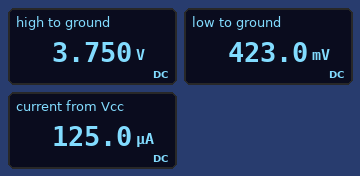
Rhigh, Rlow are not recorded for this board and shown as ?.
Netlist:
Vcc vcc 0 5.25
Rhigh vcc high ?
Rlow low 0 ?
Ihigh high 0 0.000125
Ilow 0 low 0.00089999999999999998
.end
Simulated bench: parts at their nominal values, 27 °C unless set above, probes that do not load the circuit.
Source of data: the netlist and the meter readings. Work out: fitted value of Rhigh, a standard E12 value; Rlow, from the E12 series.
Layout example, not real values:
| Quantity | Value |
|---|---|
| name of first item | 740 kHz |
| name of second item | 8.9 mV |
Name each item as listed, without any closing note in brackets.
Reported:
| Quantity | Value |
|---|---|
| fitted value of Rhigh, a standard E12 value | 12 kΩ |
| Rlow, from the E12 series | 470 Ω |
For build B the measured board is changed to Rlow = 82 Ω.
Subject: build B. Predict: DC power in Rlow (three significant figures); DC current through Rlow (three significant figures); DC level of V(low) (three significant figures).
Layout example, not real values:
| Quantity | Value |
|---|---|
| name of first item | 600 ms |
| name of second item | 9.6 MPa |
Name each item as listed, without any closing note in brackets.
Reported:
| Quantity | Value |
|---|---|
| DC power in Rlow | 66.4 µW |
| DC current through Rlow | 900 µA |
| DC level of V(low) | 73.8 mV |
